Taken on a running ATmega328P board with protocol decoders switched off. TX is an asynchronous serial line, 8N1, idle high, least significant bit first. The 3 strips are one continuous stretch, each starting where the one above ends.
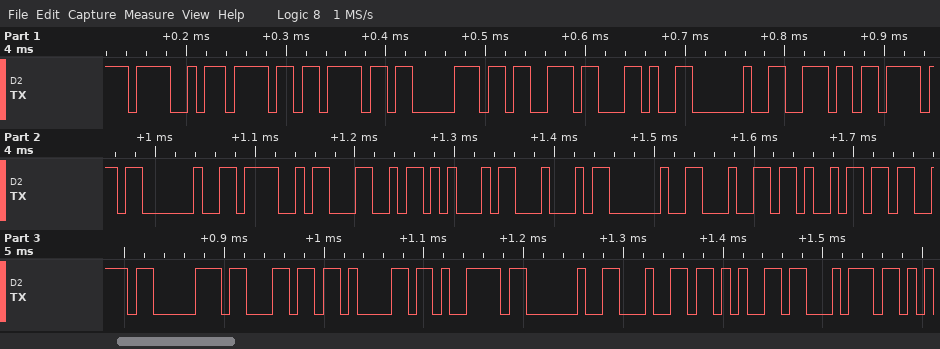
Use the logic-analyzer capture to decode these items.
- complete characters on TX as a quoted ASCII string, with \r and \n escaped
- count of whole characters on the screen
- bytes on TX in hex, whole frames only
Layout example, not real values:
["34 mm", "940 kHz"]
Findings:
["\"Ooops, no OLED display det\"", "26", "0x4F 0x6F 0x6F 0x70 0x73 0x2C 0x20 0x6E 0x6F 0x20 0x4F 0x4C 0x45 0x44 0x20 0x64 0x69 0x73 0x70 0x6C 0x61 0x79 0x20 0x64 0x65 0x74"]
